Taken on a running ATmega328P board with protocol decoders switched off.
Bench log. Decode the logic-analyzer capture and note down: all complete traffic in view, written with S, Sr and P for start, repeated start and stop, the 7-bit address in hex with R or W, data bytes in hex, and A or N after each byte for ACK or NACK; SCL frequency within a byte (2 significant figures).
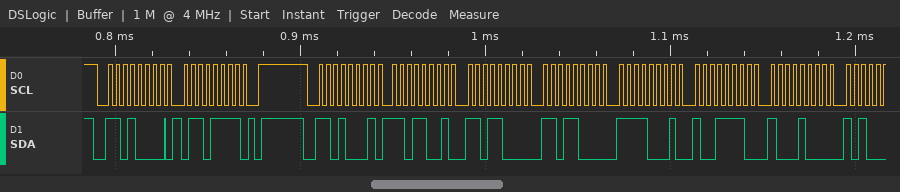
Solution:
S 68W A 6F A P S 68R A D9 A D8 A D8 A F1 A 9E A 88 A
250 kHz
